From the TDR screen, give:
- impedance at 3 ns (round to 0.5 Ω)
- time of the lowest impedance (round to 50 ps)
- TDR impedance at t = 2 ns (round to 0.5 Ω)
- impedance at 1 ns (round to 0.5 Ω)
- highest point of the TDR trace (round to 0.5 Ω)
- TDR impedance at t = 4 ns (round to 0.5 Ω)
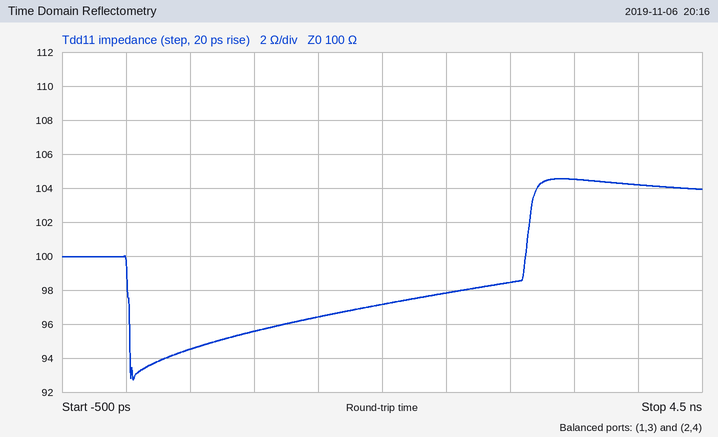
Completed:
98.5 Ω
50 ps
97.0 Ω
95.5 Ω
104.5 Ω
104.0 Ω
